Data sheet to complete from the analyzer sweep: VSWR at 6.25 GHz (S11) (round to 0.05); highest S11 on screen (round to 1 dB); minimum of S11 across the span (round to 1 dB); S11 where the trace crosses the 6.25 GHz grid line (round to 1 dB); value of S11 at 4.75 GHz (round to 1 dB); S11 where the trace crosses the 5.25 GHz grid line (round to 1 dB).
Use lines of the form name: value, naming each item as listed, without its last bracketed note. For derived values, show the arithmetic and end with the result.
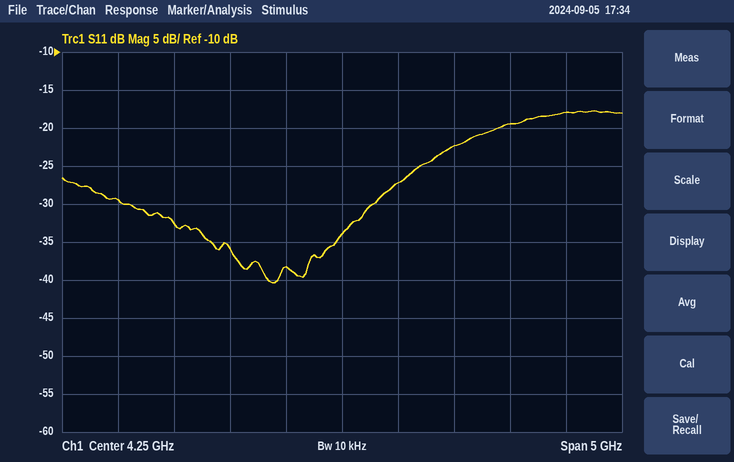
VSWR at 6.25 GHz (S11): |Γ| = 10^(-18/20) = 0.1259; VSWR = (1 + 0.1259)/(1 − 0.1259) ≈ 1.29, so 1.30 to the nearest 0.05
highest S11 on screen: -18 dB
minimum of S11 across the span: -40 dB
S11 where the trace crosses the 6.25 GHz grid line: -18 dB
value of S11 at 4.75 GHz: -27 dB
S11 where the trace crosses the 5.25 GHz grid line: -22 dB
